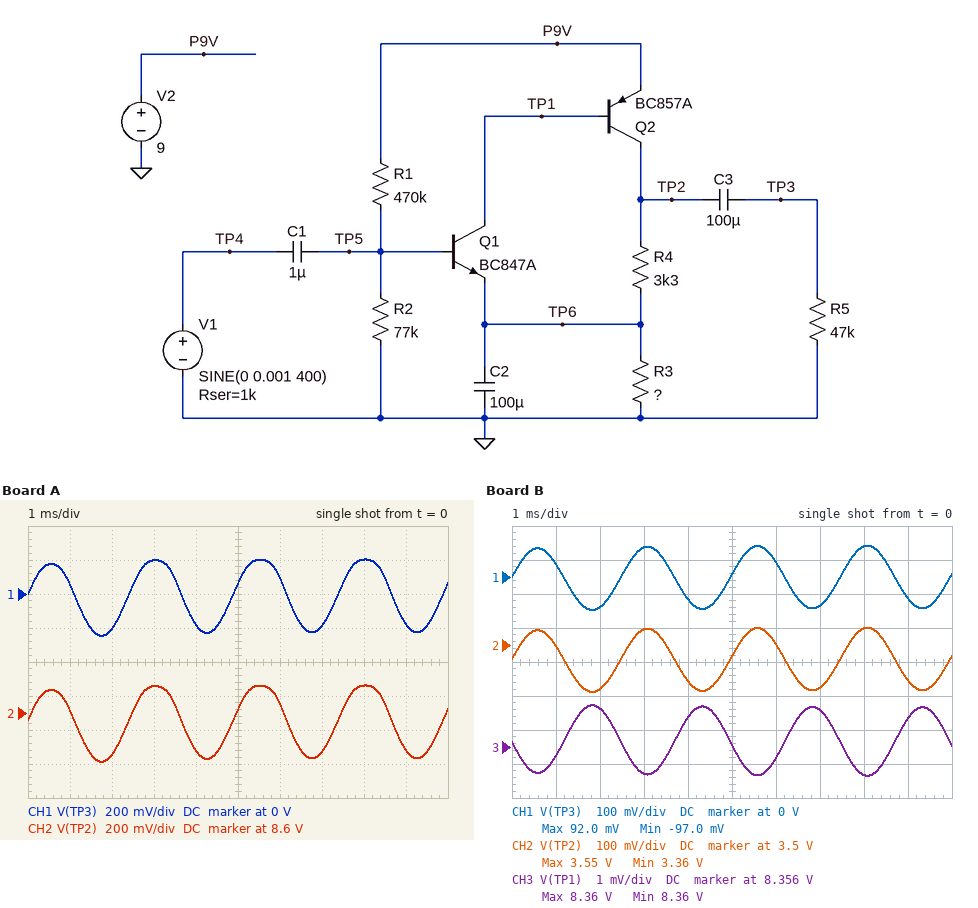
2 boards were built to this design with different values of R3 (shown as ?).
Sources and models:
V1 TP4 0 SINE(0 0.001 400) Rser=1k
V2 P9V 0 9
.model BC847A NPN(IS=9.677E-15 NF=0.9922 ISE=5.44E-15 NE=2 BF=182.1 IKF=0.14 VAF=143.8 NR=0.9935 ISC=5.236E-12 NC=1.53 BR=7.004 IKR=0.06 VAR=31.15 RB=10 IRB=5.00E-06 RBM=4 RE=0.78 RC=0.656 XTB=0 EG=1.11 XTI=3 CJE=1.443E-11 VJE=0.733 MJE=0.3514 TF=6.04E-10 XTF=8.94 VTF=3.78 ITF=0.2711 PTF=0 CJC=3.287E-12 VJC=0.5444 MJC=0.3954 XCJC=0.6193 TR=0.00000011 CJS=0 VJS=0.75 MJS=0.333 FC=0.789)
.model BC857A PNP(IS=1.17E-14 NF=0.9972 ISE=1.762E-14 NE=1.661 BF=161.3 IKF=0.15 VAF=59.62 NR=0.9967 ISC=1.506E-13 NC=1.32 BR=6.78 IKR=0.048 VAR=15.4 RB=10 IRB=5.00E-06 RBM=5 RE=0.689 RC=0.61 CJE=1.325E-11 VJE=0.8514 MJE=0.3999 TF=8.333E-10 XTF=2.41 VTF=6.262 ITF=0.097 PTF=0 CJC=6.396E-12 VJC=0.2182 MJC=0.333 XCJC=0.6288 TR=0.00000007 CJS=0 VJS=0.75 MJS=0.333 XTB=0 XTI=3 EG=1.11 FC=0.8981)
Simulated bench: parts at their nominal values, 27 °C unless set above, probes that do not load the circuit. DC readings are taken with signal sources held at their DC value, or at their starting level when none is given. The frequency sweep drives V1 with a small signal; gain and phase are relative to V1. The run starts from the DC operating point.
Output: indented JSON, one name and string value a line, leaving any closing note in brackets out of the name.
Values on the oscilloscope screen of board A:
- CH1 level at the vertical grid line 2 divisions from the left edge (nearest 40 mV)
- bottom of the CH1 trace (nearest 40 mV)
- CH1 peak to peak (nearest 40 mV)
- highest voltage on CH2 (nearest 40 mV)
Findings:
{
  "CH1 level at the vertical grid line 2 divisions from the left edge": "-200 mV",
  "bottom of the CH1 trace": "-240 mV",
  "CH1 peak to peak": "440 mV",
  "highest voltage on CH2": "8.76 V"
}
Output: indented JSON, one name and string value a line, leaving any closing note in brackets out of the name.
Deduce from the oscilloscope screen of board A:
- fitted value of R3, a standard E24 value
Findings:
{
  "fitted value of R3, a standard E24 value": "300 Ω"
}
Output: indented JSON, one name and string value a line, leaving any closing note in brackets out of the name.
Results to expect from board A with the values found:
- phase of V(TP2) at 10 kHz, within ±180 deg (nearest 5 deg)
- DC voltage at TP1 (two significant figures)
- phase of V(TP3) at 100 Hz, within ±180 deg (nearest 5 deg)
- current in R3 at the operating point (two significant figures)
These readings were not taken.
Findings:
{
  "phase of V(TP2) at 10 kHz, within ±180 deg": "-30 deg",
  "DC voltage at TP1": "8.3 V",
  "phase of V(TP3) at 100 Hz, within ±180 deg": "50 deg",
  "current in R3 at the operating point": "2.4 mA"
}
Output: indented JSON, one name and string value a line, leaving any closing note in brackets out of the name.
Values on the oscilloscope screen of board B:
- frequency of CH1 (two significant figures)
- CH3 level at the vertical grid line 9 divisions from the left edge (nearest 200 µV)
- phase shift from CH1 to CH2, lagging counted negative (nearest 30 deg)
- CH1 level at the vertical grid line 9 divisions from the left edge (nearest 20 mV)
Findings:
{
  "frequency of CH1": "400 Hz",
  "CH3 level at the vertical grid line 9 divisions from the left edge": "8.3568 V",
  "phase shift from CH1 to CH2, lagging counted negative": "0 deg",
  "CH1 level at the vertical grid line 9 divisions from the left edge": "-60 mV"
}
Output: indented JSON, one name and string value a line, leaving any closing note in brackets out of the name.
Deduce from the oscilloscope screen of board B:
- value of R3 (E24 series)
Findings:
{
  "value of R3": "910 Ω"
}
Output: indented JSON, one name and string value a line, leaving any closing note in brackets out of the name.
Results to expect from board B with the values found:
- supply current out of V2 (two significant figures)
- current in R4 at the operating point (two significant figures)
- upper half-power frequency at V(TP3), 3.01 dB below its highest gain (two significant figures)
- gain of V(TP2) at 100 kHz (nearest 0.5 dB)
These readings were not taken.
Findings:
{
  "supply current out of V2": "840 µA",
  "current in R4 at the operating point": "820 µA",
  "upper half-power frequency at V(TP3), 3.01 dB below its highest gain": "120 kHz",
  "gain of V(TP2) at 100 kHz": "37.0 dB"
}
